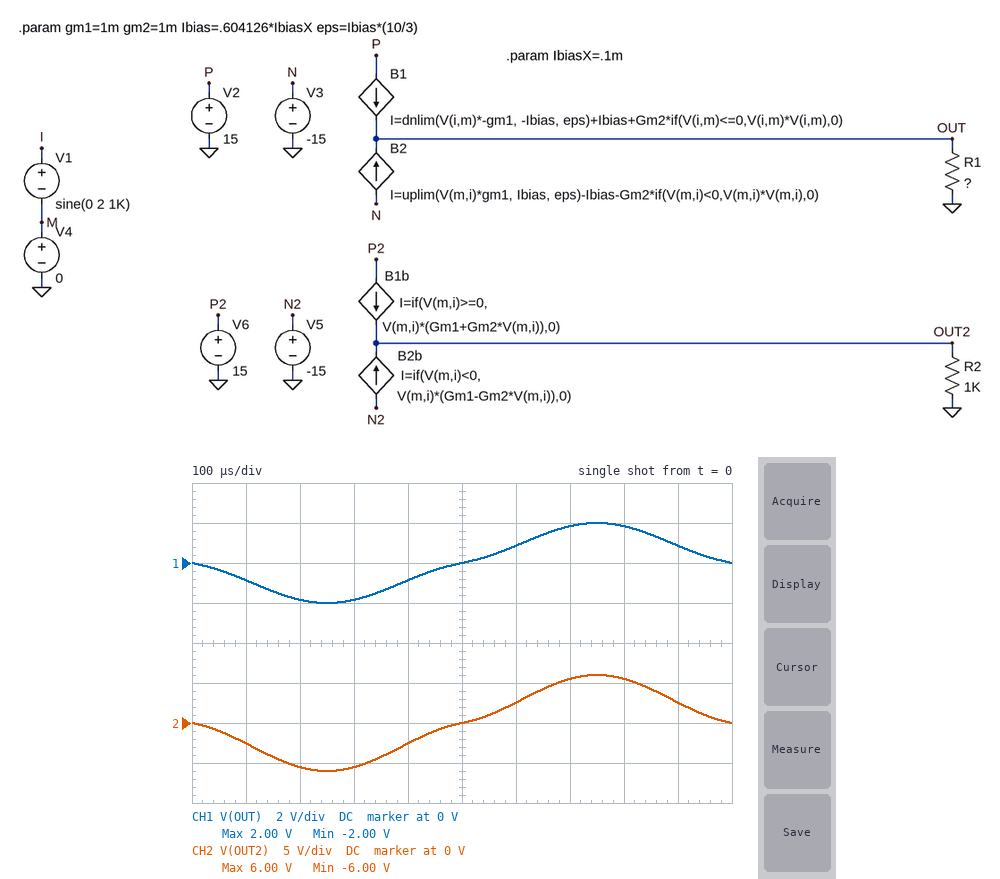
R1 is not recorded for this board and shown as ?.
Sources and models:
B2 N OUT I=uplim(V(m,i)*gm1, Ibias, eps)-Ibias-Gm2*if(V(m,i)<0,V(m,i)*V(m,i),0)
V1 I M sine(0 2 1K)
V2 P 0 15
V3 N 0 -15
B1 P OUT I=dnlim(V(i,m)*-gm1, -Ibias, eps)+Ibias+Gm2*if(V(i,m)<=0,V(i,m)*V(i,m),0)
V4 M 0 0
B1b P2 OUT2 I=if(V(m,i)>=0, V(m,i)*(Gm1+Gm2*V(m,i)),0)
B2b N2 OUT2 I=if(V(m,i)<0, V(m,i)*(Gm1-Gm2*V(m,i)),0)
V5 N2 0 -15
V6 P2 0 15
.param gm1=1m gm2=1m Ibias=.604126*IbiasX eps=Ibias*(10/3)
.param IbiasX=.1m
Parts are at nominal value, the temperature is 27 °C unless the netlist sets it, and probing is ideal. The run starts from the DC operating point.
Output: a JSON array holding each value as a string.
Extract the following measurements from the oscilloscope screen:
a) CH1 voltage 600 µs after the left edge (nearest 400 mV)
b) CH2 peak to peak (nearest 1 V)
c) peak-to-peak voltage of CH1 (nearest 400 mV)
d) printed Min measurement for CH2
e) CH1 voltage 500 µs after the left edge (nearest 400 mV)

["800 mV", "12 V", "4.0 V", "-6.00 V", "0 V"]
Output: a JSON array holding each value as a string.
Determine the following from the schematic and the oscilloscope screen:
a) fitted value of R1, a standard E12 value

["330 Ω"]
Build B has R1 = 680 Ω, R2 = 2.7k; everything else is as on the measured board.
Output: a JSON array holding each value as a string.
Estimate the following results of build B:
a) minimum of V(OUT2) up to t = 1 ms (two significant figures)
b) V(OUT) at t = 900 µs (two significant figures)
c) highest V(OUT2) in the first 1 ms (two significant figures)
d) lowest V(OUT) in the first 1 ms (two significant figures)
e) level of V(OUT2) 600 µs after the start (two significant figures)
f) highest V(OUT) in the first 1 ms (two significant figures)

["-16 V", "1.8 V", "16 V", "-4.1 V", "6.9 V", "4.1 V"]
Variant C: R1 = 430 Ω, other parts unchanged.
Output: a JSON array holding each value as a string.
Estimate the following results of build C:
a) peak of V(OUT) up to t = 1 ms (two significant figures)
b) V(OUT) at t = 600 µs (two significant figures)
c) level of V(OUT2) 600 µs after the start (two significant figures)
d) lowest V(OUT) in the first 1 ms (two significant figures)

["2.6 V", "1.1 V", "2.6 V", "-2.6 V"]
